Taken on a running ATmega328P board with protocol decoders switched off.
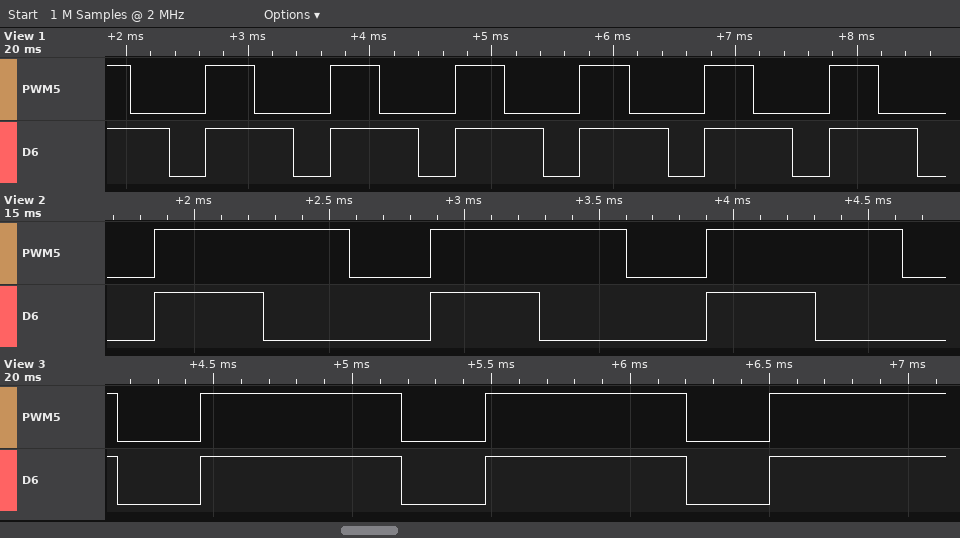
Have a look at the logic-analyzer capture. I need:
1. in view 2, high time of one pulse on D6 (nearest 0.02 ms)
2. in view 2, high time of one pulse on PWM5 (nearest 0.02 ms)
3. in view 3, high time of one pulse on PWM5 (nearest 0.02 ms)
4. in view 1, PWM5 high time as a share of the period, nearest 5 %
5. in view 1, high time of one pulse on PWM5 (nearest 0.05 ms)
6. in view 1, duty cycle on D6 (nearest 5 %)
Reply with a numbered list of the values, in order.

1. 0.40 ms
2. 0.72 ms
3. 0.72 ms
4. 40 %
5. 0.40 ms
6. 70 %
